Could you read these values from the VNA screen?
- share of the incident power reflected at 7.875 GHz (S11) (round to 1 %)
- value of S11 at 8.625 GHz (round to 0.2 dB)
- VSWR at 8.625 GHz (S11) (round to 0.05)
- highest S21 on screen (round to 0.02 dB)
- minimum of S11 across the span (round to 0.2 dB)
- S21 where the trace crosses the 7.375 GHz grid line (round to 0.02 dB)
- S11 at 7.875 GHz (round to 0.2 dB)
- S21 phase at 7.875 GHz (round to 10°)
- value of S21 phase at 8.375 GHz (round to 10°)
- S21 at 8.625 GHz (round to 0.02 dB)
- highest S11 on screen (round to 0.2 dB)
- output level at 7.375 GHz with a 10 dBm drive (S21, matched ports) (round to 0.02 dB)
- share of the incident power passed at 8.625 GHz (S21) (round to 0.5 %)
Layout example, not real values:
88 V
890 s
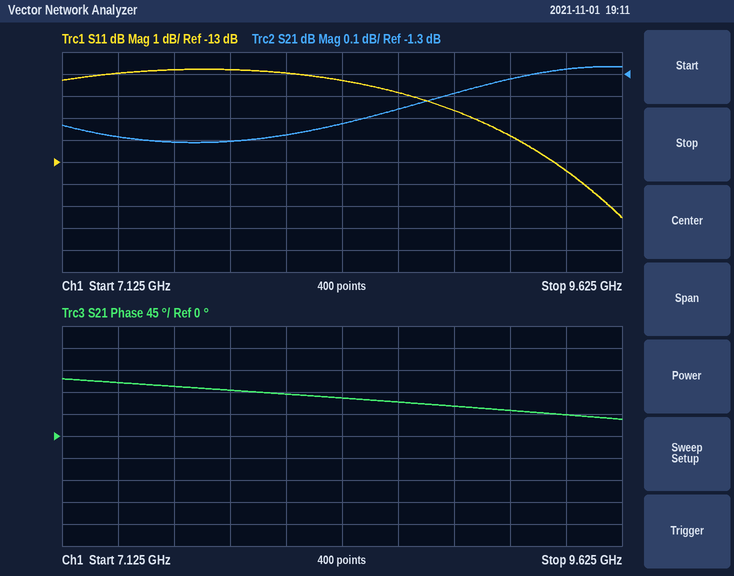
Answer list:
13 %
-9.8 dB
1.95
-1.26 dB
-15.6 dB
-1.58 dB
-8.8 dB
90°
80°
-1.46 dB
-8.8 dB
8.42 dBm
71.5 %
